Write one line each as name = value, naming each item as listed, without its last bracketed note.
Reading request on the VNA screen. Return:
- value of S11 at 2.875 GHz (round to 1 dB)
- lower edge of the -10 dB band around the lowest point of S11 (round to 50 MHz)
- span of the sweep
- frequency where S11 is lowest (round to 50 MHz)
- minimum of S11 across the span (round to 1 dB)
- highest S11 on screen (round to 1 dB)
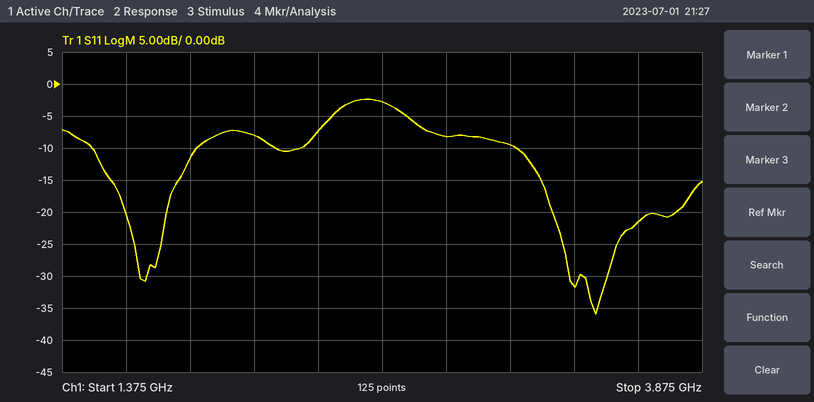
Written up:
value of S11 at 2.875 GHz = -8 dB
lower edge of the -10 dB band around the lowest point of S11 = 3.15 GHz
span of the sweep = 2.5 GHz
frequency where S11 is lowest = 3.45 GHz
minimum of S11 across the span = -36 dB
highest S11 on screen = -2 dB
